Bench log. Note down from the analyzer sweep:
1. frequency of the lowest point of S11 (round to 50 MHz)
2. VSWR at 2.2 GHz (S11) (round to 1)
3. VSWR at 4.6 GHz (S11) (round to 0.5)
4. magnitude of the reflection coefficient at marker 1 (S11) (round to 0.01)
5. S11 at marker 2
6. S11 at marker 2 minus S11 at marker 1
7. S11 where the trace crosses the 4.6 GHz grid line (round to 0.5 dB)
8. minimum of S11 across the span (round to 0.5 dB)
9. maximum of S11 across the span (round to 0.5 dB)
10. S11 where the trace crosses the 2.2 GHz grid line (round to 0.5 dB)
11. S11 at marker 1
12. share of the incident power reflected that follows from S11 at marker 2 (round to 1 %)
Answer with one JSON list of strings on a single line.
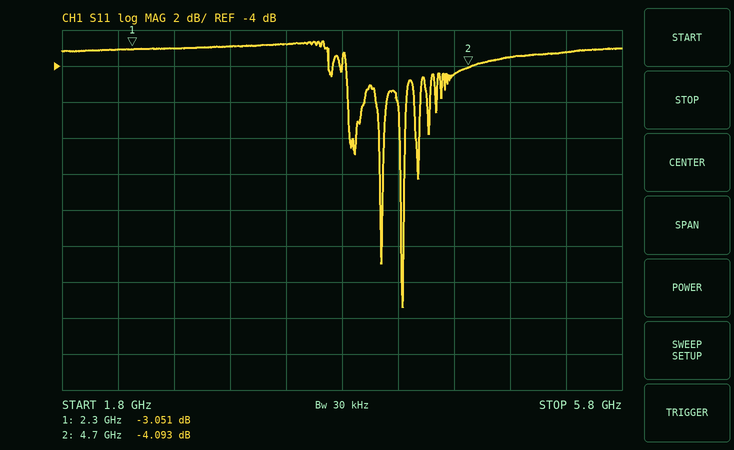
["4.25 GHz", "6", "4.0", "0.70", "-4.093 dB", "-1.042 dB", "-4.5 dB", "-17.5 dB", "-2.5 dB", "-3.0 dB", "-3.051 dB", "39 %"]
